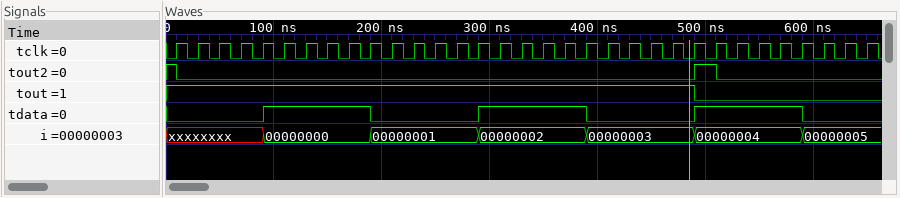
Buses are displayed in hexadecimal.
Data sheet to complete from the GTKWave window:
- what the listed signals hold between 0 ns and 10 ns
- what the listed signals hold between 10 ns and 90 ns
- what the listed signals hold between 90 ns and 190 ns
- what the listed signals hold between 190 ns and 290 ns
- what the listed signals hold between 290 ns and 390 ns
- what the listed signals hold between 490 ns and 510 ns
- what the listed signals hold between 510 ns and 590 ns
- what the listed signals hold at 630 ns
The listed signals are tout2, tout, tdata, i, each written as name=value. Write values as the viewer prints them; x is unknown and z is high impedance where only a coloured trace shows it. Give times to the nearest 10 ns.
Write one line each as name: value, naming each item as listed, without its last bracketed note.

what the listed signals hold between 0 ns and 10 ns: tout2=1, tout=1, tdata=0, i=xxxxxxxx
what the listed signals hold between 10 ns and 90 ns: tout2=0, tout=1, tdata=0, i=xxxxxxxx
what the listed signals hold between 90 ns and 190 ns: tout2=0, tout=1, tdata=1, i=00000000
what the listed signals hold between 190 ns and 290 ns: tout2=0, tout=1, tdata=0, i=00000001
what the listed signals hold between 290 ns and 390 ns: tout2=0, tout=1, tdata=1, i=00000002
what the listed signals hold between 490 ns and 510 ns: tout2=1, tout=0, tdata=1, i=00000004
what the listed signals hold between 510 ns and 590 ns: tout2=0, tout=0, tdata=1, i=00000004
what the listed signals hold at 630 ns: tout2=0, tout=0, tdata=0, i=00000005
